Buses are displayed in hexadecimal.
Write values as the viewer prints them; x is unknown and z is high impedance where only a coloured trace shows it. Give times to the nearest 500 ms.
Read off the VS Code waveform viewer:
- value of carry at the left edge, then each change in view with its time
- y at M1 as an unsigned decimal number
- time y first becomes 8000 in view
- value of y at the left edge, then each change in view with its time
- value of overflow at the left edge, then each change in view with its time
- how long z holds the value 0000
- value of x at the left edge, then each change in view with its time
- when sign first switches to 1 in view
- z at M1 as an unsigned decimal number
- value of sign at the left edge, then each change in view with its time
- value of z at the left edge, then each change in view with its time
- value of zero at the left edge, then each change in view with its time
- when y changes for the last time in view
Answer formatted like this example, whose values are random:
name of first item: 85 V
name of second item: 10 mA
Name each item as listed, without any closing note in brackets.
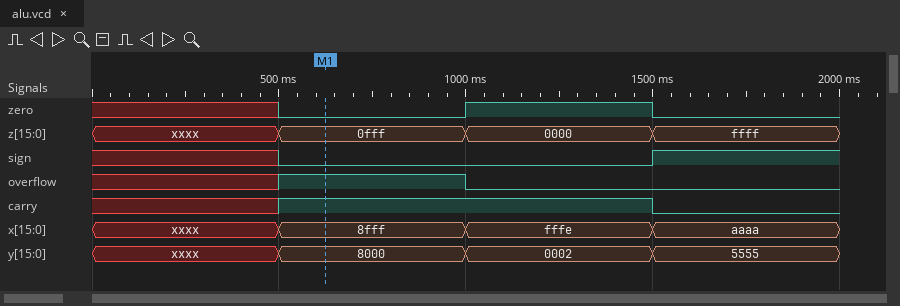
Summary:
value of carry at the left edge, then each change in view with its time: x, 1 at 500 ms, 0 at 1500 ms
y at M1 as an unsigned decimal number: 32768
time y first becomes 8000 in view: 500 ms
value of y at the left edge, then each change in view with its time: xxxx, 8000 at 500 ms, 0002 at 1000 ms, 5555 at 1500 ms
value of overflow at the left edge, then each change in view with its time: x, 1 at 500 ms, 0 at 1000 ms
how long z holds the value 0000: 500 ms
value of x at the left edge, then each change in view with its time: xxxx, 8fff at 500 ms, fffe at 1000 ms, aaaa at 1500 ms
when sign first switches to 1 in view: 1500 ms
z at M1 as an unsigned decimal number: 4095
value of sign at the left edge, then each change in view with its time: x, 0 at 500 ms, 1 at 1500 ms
value of z at the left edge, then each change in view with its time: xxxx, 0fff at 500 ms, 0000 at 1000 ms, ffff at 1500 ms
value of zero at the left edge, then each change in view with its time: x, 0 at 500 ms, 1 at 1000 ms, 0 at 1500 ms
when y changes for the last time in view: 1500 ms
